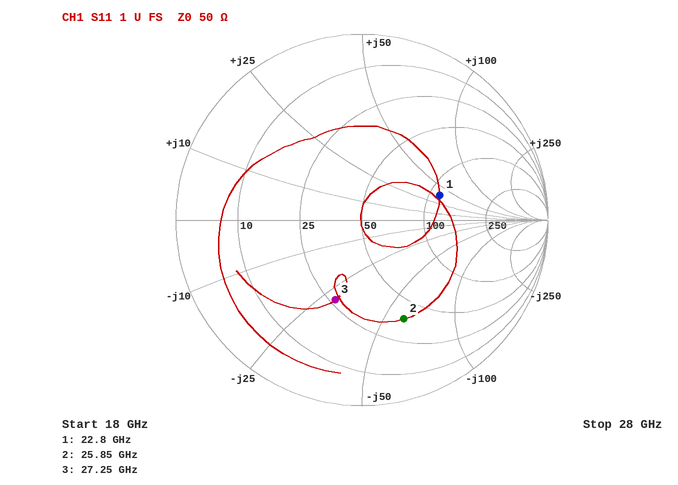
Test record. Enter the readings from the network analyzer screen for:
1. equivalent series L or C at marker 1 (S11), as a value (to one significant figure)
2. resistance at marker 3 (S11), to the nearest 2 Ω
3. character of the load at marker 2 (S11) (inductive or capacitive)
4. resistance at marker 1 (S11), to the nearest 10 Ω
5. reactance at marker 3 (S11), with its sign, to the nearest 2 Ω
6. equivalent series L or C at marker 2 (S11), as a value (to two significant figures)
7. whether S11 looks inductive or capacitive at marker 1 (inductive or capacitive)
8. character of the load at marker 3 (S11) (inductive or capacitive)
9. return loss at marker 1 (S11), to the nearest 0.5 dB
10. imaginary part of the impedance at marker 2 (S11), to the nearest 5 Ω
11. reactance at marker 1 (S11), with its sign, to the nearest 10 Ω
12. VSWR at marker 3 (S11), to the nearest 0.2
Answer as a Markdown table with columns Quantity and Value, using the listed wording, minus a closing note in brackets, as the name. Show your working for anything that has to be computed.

| Quantity | Value |
|---|---|
| equivalent series L or C at marker 1 (S11), as a value | L = 40 Ω/(2π × 22.8 GHz) ≈ 279 pH, so 300 pH to one significant figure |
| resistance at marker 3 (S11), to the nearest 2 Ω | 26 Ω |
| character of the load at marker 2 (S11) | capacitive |
| resistance at marker 1 (S11), to the nearest 10 Ω | 110 Ω |
| reactance at marker 3 (S11), with its sign, to the nearest 2 Ω | -28 Ω |
| equivalent series L or C at marker 2 (S11), as a value | C = 1/(2π × 25.85 GHz × 60 Ω) ≈ 103 fF, so 100 fF to two significant figures |
| whether S11 looks inductive or capacitive at marker 1 | inductive |
| character of the load at marker 3 (S11) | capacitive |
| return loss at marker 1 (S11), to the nearest 0.5 dB | 7.0 dB |
| imaginary part of the impedance at marker 2 (S11), to the nearest 5 Ω | -60 Ω |
| reactance at marker 1 (S11), with its sign, to the nearest 10 Ω | +40 Ω |
| VSWR at marker 3 (S11), to the nearest 0.2 | 2.6 |
